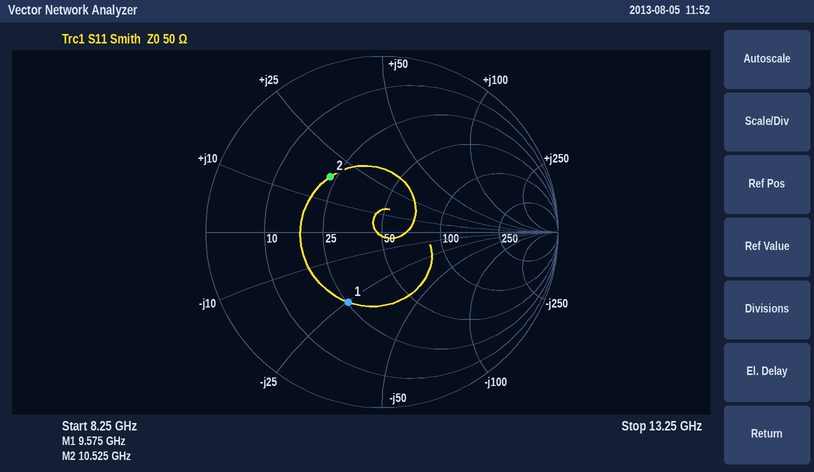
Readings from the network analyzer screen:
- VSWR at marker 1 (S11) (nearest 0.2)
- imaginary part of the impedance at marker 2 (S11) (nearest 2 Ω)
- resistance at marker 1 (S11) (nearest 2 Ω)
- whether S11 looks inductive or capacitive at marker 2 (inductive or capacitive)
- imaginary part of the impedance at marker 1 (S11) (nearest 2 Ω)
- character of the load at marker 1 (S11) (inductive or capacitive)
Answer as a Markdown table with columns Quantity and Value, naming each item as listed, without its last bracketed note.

| Quantity | Value |
|---|---|
| VSWR at marker 1 (S11) | 2.6 |
| imaginary part of the impedance at marker 2 (S11) | +18 Ω |
| resistance at marker 1 (S11) | 26 Ω |
| whether S11 looks inductive or capacitive at marker 2 | inductive |
| imaginary part of the impedance at marker 1 (S11) | -26 Ω |
| character of the load at marker 1 (S11) | capacitive |
